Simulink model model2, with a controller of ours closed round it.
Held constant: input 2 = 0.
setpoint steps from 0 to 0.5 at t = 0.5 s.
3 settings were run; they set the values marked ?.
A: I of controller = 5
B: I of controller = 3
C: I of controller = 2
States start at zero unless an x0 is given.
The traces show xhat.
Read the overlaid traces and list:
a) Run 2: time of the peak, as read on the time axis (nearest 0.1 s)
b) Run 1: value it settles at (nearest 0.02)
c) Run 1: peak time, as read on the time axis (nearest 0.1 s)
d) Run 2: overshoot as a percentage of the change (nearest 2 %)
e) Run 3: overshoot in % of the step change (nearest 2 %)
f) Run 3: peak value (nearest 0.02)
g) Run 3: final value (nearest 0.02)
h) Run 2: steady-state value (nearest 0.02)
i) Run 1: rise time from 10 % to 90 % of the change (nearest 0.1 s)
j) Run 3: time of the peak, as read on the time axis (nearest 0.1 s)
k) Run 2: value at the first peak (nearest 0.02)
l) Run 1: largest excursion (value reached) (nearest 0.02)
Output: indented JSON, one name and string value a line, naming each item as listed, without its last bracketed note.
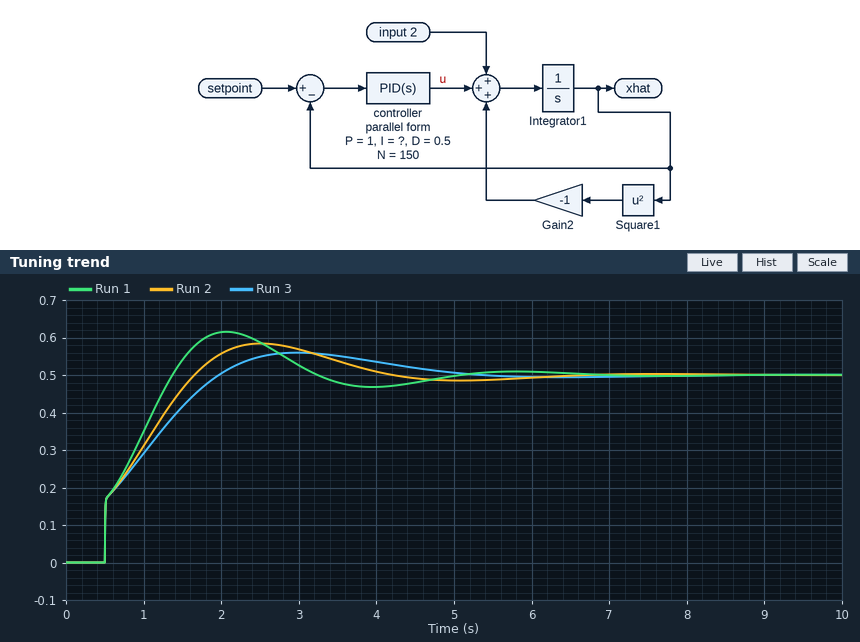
{
  "Run 2: time of the peak, as read on the time axis": "2.5 s",
  "Run 1: value it settles at": "0.50",
  "Run 1: peak time, as read on the time axis": "2.1 s",
  "Run 2: overshoot as a percentage of the change": "16 %",
  "Run 3: overshoot in % of the step change": "12 %",
  "Run 3: peak value": "0.56",
  "Run 3: final value": "0.50",
  "Run 2: steady-state value": "0.50",
  "Run 1: rise time from 10 % to 90 % of the change": "0.7 s",
  "Run 3: time of the peak, as read on the time axis": "3.0 s",
  "Run 2: value at the first peak": "0.58",
  "Run 1: largest excursion (value reached)": "0.62"
}
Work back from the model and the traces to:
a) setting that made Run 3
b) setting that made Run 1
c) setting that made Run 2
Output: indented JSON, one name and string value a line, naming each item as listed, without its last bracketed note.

{
  "setting that made Run 3": "C",
  "setting that made Run 1": "A",
  "setting that made Run 2": "B"
}
